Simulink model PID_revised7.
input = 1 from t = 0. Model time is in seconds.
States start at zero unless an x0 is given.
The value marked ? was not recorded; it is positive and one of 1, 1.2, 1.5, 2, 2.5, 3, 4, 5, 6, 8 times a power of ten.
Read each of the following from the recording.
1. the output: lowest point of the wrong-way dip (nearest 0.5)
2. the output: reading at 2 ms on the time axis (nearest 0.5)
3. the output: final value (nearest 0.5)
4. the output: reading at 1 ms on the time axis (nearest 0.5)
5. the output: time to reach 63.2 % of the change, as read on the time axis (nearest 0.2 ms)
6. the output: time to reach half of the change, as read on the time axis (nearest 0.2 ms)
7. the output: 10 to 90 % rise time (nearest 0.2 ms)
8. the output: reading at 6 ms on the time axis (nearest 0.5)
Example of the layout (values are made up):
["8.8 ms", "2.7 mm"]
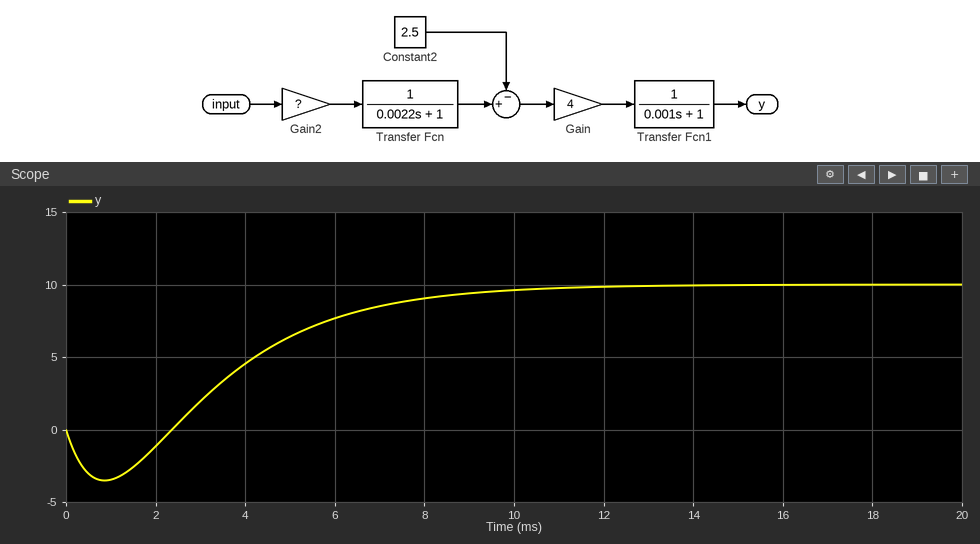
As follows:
["-3.5", "-1.0", "10.0", "-3.5", "5.0 ms", "4.2 ms", "5.2 ms", "7.5"]
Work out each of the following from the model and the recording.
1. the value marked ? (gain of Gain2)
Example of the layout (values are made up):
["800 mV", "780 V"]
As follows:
["5"]
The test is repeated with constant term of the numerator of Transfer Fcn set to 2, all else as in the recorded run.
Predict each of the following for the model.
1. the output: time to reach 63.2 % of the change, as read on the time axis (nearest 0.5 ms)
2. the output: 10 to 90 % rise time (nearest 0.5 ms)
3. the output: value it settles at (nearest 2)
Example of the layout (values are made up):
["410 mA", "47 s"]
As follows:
["4.0 ms", "5.5 ms", "30"]
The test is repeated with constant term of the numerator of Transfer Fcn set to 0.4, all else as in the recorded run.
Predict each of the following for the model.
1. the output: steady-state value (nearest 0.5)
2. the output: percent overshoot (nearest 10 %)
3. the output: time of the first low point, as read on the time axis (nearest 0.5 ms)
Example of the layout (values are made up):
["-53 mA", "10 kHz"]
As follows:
["-2.0", "190 %", "1.5 ms"]
